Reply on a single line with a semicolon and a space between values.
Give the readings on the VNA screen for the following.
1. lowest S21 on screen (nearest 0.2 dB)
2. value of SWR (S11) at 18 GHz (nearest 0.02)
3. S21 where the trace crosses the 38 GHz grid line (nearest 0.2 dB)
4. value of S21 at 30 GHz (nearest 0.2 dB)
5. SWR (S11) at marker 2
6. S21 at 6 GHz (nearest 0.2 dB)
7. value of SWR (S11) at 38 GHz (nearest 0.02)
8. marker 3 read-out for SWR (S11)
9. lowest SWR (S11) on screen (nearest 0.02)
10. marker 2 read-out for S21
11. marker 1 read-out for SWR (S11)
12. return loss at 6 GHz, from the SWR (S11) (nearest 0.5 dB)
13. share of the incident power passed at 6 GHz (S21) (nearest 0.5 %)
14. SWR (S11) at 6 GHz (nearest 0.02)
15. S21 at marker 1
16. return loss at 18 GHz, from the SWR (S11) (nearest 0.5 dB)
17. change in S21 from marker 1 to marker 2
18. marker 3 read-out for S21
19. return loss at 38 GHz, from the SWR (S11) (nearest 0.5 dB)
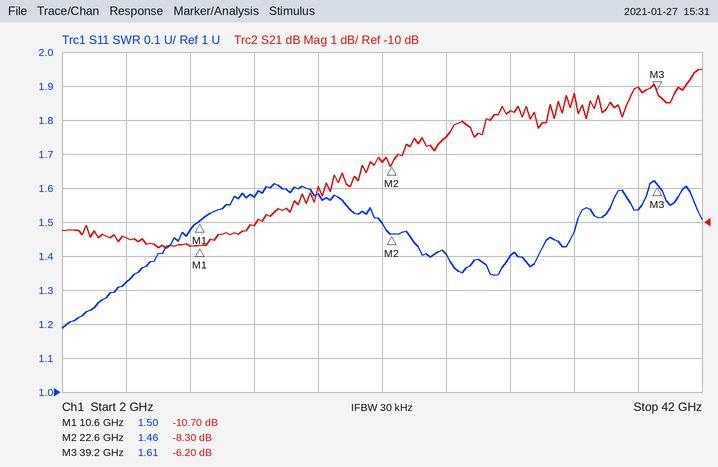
-10.8 dB; 1.58; -6.0 dB; -6.8 dB; 1.46; -10.4 dB; 1.54; 1.61; 1.18; -8.30 dB; 1.50; 17.0 dB; 9.0 %; 1.32; -10.70 dB; 13.0 dB; 2.40 dB; -6.20 dB; 13.5 dB
